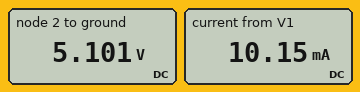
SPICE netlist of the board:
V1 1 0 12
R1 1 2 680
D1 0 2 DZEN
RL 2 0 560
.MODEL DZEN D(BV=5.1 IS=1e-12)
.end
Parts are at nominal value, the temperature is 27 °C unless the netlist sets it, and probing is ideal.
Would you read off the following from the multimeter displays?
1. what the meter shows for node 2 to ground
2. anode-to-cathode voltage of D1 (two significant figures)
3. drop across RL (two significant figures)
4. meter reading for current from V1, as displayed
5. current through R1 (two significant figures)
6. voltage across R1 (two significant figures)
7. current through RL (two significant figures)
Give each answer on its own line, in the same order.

5.101 V
-5.1 V
5.1 V
10.15 mA
10 mA
6.9 V
9.1 mA
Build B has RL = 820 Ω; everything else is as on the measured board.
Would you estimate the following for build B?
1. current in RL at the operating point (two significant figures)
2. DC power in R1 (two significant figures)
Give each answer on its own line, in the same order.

6.3 mA
69 mW
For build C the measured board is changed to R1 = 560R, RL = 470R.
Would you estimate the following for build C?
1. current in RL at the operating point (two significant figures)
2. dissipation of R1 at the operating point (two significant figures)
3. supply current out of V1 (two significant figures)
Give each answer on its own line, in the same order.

11 mA
85 mW
12 mA
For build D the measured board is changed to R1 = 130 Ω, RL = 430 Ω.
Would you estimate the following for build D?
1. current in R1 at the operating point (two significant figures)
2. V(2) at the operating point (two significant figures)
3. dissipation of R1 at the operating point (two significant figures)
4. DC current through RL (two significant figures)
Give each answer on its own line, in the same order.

52 mA
5.2 V
360 mW
12 mA
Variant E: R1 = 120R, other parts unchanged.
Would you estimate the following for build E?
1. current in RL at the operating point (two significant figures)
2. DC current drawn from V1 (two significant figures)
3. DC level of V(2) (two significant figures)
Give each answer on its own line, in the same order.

9.3 mA
57 mA
5.2 V
